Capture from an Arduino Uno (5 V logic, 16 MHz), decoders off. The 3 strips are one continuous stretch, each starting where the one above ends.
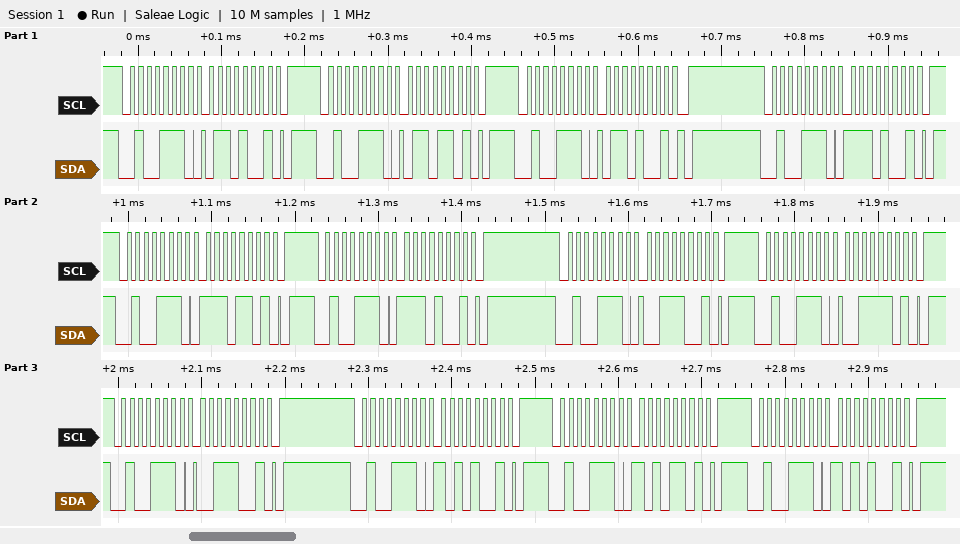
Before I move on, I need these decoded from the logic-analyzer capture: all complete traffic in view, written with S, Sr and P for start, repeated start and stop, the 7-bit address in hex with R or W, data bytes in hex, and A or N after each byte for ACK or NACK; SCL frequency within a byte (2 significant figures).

S 27W A 69 A P S 27W A 6D A P S 27W A 69 A P S 27W A E9 A P S 27W A ED A P S 27W A E9 A P S 27W A 39 A P S 27W A 3D A P S 27W A 39 A P S 27W A A9 A P S 27W A AD A P S 27W A A9 A P
100 kHz
